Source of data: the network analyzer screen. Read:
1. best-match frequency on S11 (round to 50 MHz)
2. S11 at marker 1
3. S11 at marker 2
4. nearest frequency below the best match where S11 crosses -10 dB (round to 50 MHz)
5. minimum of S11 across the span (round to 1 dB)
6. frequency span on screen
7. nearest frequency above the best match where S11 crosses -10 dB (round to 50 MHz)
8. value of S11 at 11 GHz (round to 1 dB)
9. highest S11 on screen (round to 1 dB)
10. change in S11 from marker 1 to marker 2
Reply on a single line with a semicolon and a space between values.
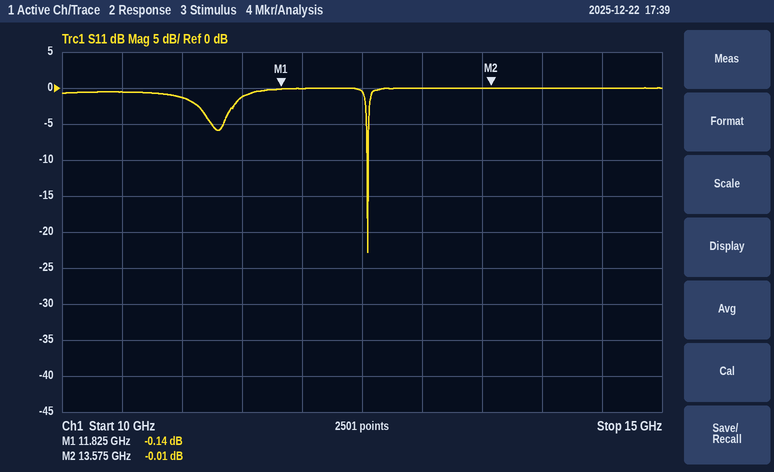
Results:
12.55 GHz; -0.14 dB; -0.01 dB; 12.55 GHz; -23 dB; 5 GHz; 12.55 GHz; -1 dB; 0 dB; 0.13 dB
